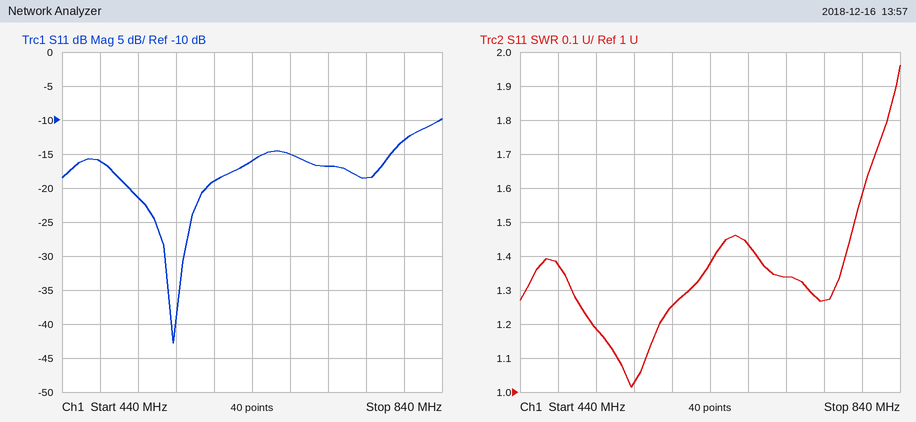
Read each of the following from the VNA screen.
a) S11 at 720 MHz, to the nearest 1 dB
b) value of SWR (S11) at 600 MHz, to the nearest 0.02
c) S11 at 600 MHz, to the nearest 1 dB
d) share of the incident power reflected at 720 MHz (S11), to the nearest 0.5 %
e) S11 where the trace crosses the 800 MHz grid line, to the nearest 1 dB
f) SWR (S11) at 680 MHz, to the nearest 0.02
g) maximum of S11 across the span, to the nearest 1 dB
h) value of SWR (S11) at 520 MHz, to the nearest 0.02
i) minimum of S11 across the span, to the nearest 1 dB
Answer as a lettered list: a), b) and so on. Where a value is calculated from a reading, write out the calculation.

a) -17 dB
b) 1.26
c) -19 dB
d) 10^(-17/10) ≈ 2.0 %
e) -13 dB
f) 1.44
g) -10 dB
h) 1.18
i) -43 dB
